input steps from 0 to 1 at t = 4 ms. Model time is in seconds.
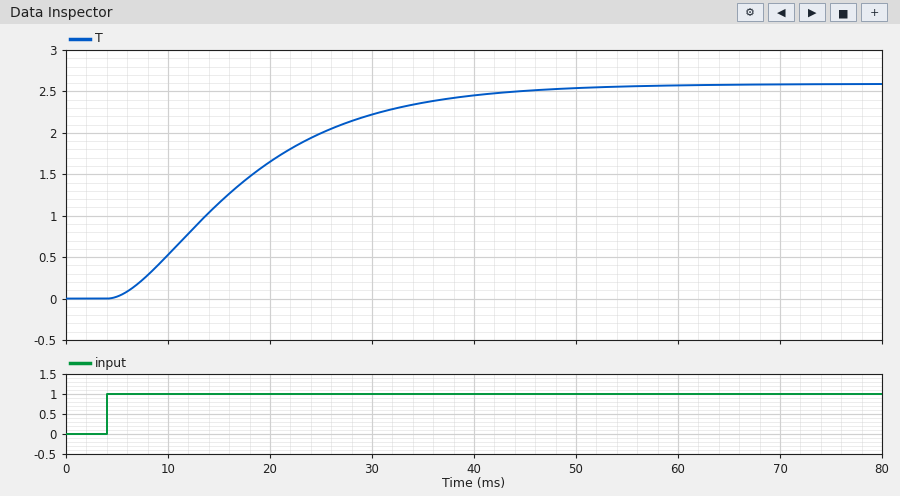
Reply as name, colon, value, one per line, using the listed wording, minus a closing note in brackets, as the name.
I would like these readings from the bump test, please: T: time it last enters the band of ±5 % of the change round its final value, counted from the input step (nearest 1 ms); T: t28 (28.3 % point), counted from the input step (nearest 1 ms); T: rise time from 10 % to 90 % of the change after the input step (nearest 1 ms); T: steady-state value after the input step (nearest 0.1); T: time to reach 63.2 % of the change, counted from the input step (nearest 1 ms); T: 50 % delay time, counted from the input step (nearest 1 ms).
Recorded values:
T: time it last enters the band of ±5 % of the change round its final value, counted from the input step: 37 ms
T: t28 (28.3 % point), counted from the input step: 8 ms
T: rise time from 10 % to 90 % of the change after the input step: 26 ms
T: steady-state value after the input step: 2.6
T: time to reach 63.2 % of the change, counted from the input step: 16 ms
T: 50 % delay time, counted from the input step: 12 ms
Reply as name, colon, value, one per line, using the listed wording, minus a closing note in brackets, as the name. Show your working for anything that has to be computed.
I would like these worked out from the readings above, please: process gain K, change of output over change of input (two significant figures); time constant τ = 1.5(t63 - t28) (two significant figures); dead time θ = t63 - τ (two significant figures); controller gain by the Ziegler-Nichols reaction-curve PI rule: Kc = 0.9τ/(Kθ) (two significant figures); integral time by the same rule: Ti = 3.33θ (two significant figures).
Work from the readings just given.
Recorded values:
process gain K, change of output over change of input: (2.6 - 0) / 1 = 2.6
time constant τ = 1.5(t63 - t28): 1.5 × (16 - 8) = 12 ms
dead time θ = t63 - τ: 16 - 12 = 4.0 ms
controller gain by the Ziegler-Nichols reaction-curve PI rule: Kc = 0.9τ/(Kθ): 0.9 × 12 / (2.6 × 4) = 1.0
integral time by the same rule: Ti = 3.33θ: 3.33 × 4 = 13 ms
